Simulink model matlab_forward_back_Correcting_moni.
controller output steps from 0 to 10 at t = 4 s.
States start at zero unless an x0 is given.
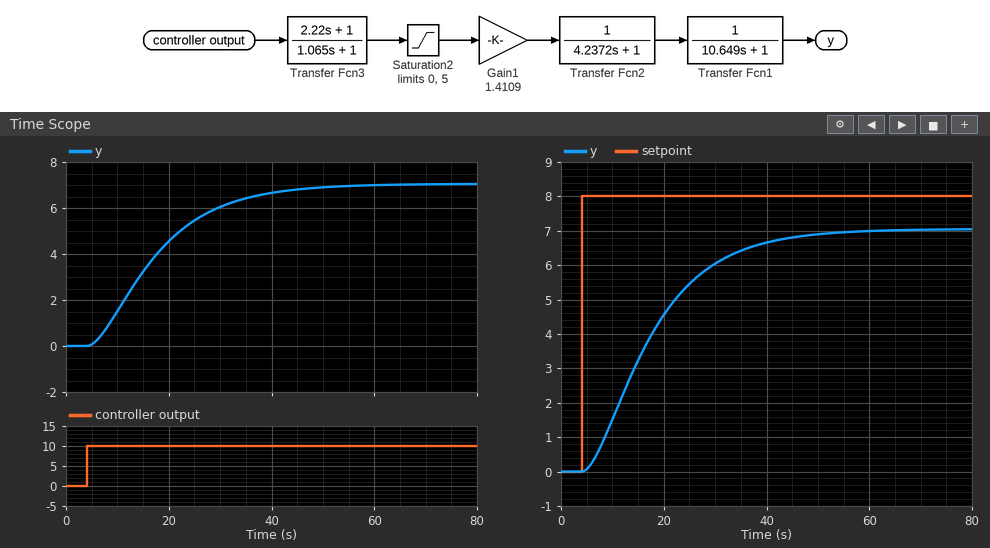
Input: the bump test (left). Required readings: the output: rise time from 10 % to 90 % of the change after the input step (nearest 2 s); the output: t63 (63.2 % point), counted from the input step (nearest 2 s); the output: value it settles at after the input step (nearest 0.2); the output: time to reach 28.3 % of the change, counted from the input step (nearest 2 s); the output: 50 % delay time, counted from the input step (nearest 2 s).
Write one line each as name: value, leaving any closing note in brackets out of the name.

the output: rise time from 10 % to 90 % of the change after the input step: 26 s
the output: t63 (63.2 % point), counted from the input step: 16 s
the output: value it settles at after the input step: 7.0
the output: time to reach 28.3 % of the change, counted from the input step: 8 s
the output: 50 % delay time, counted from the input step: 12 s
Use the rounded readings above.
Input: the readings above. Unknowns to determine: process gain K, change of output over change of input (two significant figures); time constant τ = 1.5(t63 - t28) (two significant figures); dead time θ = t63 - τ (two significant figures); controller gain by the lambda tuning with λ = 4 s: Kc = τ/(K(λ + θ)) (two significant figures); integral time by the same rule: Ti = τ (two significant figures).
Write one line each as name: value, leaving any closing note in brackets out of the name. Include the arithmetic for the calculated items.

process gain K, change of output over change of input: (7 - 0) / 10 = 0.70
time constant τ = 1.5(t63 - t28): 1.5 × (16 - 8) = 12 s
dead time θ = t63 - τ: 16 - 12 = 4.0 s
controller gain by the lambda tuning with λ = 4 s: Kc = τ/(K(λ + θ)): 12 / (0.7 × (4 + 4)) = 2.1
integral time by the same rule: Ti = τ: 12 s
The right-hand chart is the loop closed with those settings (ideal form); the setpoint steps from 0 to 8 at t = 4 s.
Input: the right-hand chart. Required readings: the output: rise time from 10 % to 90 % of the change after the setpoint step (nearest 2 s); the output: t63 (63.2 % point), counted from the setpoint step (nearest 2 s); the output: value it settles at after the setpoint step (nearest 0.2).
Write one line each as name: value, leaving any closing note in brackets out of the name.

the output: rise time from 10 % to 90 % of the change after the setpoint step: 26 s
the output: t63 (63.2 % point), counted from the setpoint step: 16 s
the output: value it settles at after the setpoint step: 7.0
